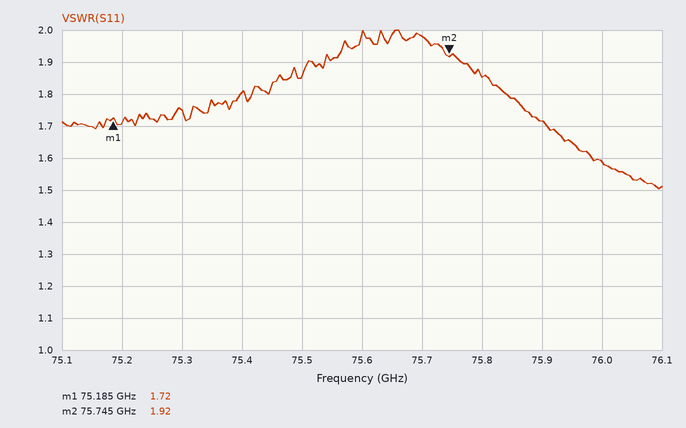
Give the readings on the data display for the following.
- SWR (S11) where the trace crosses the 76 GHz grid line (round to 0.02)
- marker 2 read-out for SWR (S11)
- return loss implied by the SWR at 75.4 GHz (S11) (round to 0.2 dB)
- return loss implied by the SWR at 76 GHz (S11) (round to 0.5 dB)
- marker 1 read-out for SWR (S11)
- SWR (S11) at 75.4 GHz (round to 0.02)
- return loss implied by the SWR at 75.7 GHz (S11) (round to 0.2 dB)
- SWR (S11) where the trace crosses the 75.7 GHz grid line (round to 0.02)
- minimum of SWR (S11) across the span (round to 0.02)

1.58
1.92
10.8 dB
13.0 dB
1.72
1.80
9.6 dB
1.98
1.50
